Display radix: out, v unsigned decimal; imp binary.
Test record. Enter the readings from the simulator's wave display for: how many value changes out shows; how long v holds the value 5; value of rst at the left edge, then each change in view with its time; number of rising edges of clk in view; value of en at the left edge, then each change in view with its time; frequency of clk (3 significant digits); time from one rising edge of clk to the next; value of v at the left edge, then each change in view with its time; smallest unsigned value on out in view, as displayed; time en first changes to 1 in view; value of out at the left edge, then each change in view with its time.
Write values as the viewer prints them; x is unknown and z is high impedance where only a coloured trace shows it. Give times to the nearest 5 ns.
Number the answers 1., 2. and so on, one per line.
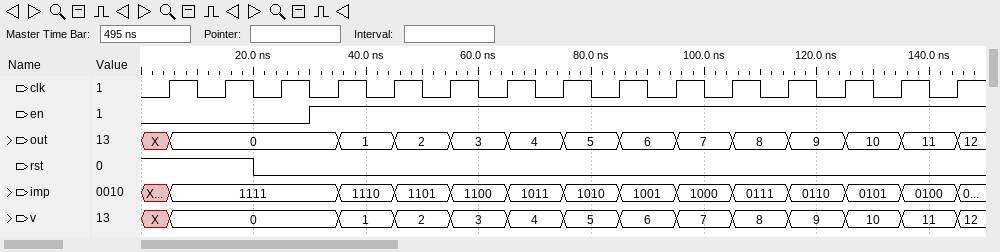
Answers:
1. 13
2. 10 ns
3. 1, 0 at 20 ns
4. 15
5. 0, 1 at 30 ns
6. 100 MHz
7. 10 ns
8. X, 0 at 5 ns, 1 at 35 ns, 2 at 45 ns, 3 at 55 ns, 4 at 65 ns, 5 at 75 ns, 6 at 85 ns, 7 at 95 ns, 8 at 105 ns, 9 at 115 ns, 10 at 125 ns, 11 at 135 ns, 12 at 145 ns
9. 0
10. 30 ns
11. X, 0 at 5 ns, 1 at 35 ns, 2 at 45 ns, 3 at 55 ns, 4 at 65 ns, 5 at 75 ns, 6 at 85 ns, 7 at 95 ns, 8 at 105 ns, 9 at 115 ns, 10 at 125 ns, 11 at 135 ns, 12 at 145 ns
